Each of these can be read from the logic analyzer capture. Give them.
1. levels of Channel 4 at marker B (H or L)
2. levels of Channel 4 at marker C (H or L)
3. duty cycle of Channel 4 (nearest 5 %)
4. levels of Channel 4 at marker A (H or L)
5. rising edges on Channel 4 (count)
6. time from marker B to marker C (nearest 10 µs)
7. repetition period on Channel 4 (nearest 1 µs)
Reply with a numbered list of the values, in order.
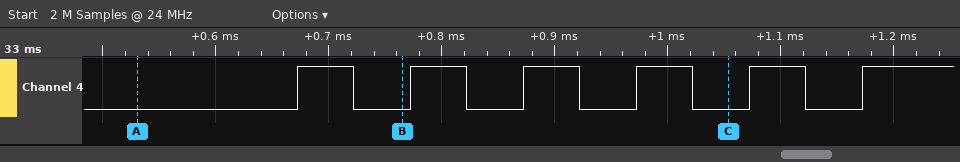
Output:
1. Channel 4=L
2. Channel 4=L
3. 50 %
4. Channel 4=L
5. 6
6. 290 µs
7. 100 µs
